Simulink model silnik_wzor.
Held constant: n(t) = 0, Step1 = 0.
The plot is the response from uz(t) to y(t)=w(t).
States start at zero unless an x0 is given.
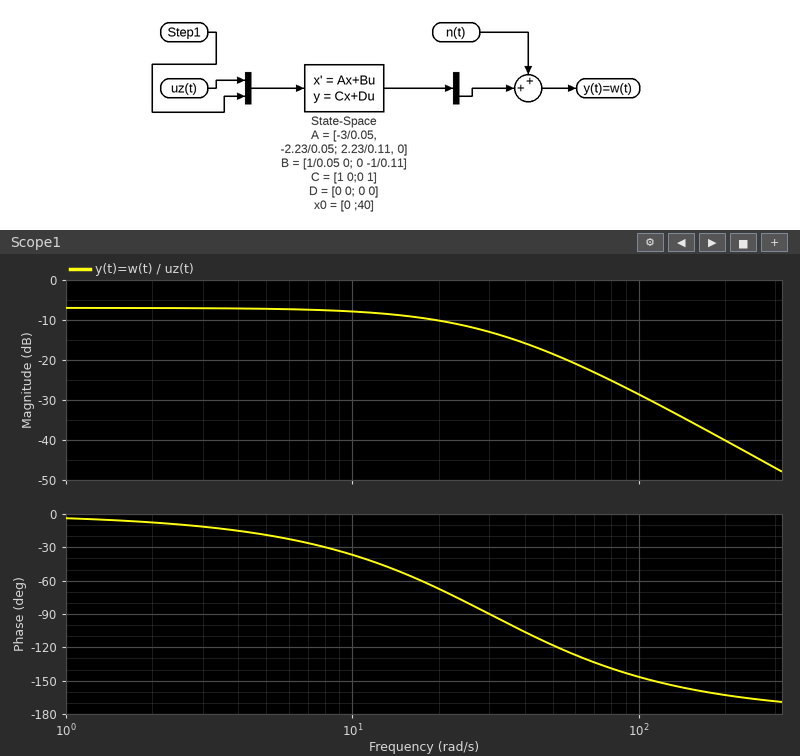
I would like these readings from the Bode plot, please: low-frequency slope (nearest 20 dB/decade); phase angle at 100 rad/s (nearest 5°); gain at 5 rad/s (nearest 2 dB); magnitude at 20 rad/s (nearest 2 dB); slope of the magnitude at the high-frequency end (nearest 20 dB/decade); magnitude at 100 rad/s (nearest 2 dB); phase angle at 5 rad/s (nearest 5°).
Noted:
0 dB/decade
-145°
-8 dB
-10 dB
-40 dB/decade
-28 dB
-20°
